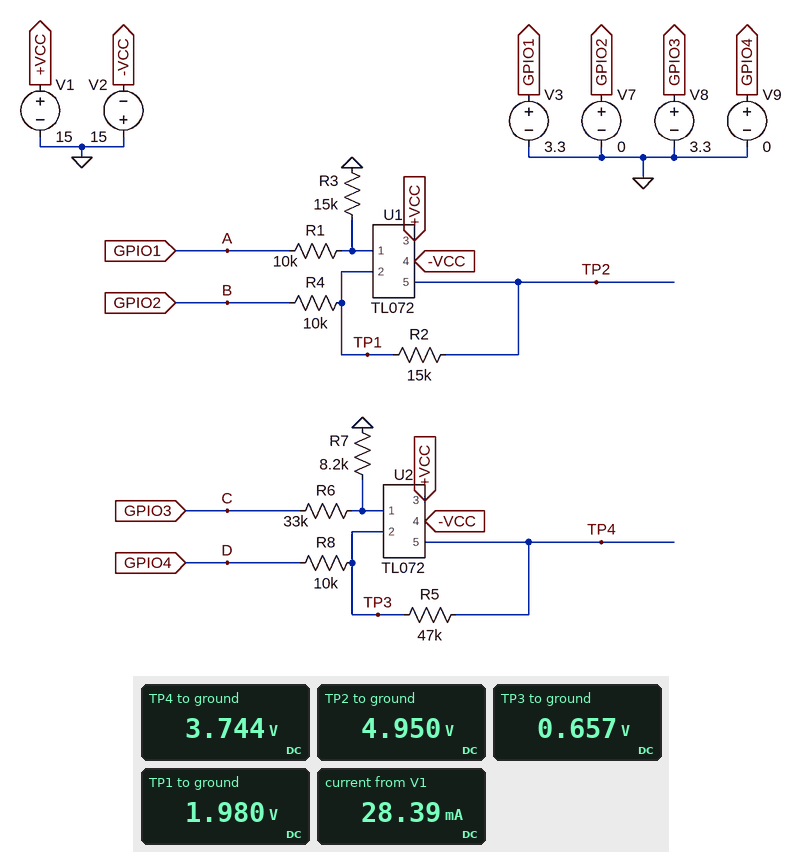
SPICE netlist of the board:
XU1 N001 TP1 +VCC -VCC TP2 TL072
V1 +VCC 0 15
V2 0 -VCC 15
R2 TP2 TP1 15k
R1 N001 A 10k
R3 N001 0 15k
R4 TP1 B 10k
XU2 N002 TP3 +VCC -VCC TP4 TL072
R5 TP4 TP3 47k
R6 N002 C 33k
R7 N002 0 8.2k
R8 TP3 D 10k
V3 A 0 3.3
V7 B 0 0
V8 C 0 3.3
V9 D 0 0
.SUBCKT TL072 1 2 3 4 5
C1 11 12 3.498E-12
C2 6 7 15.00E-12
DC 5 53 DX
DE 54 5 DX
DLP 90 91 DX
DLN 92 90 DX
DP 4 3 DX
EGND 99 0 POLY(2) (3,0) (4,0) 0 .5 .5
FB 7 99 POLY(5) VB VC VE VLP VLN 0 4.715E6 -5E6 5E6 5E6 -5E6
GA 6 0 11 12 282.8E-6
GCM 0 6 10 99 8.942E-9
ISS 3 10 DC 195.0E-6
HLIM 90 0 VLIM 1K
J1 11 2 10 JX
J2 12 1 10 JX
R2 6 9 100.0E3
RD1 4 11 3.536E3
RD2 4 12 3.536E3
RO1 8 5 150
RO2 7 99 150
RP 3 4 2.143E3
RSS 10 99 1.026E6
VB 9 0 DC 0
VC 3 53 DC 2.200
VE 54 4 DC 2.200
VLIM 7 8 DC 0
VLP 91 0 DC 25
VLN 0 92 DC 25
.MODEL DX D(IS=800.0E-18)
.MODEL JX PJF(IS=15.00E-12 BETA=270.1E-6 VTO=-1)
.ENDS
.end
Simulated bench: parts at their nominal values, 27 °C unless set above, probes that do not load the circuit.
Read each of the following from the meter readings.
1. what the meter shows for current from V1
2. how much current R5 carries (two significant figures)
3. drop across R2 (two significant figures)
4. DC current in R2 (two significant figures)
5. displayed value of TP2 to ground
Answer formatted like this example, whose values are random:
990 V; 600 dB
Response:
28.39 mA; 66 µA; 3.0 V; 200 µA; 4.950 V
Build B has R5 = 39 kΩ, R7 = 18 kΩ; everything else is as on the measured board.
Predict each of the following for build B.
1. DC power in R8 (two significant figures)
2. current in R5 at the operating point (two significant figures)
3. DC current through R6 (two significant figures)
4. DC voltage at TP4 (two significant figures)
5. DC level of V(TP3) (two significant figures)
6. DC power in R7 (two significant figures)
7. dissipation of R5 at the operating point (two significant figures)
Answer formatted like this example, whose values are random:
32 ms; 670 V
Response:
140 µW; 120 µA; 65 µA; 5.7 V; 1.2 V; 75 µW; 530 µW
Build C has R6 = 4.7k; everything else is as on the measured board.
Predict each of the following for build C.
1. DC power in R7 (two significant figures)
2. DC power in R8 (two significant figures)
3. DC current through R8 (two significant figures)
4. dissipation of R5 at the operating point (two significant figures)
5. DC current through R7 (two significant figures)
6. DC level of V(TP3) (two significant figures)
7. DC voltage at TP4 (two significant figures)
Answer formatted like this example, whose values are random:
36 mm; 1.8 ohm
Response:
540 µW; 440 µW; 210 µA; 2.1 mW; 260 µA; 2.1 V; 12 V
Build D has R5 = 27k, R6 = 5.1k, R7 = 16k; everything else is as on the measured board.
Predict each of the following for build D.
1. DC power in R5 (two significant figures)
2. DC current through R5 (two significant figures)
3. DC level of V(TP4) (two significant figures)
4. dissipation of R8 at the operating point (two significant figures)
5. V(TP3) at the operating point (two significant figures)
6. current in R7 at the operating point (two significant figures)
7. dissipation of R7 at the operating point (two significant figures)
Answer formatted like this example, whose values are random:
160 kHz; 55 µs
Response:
1.7 mW; 250 µA; 9.3 V; 630 µW; 2.5 V; 160 µA; 390 µW
